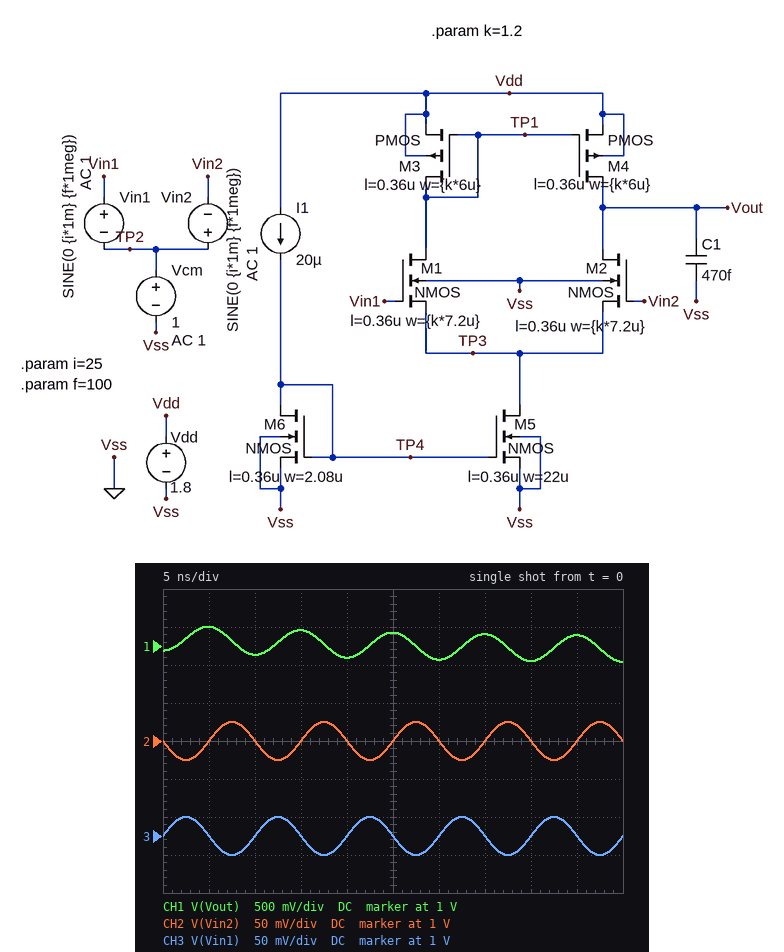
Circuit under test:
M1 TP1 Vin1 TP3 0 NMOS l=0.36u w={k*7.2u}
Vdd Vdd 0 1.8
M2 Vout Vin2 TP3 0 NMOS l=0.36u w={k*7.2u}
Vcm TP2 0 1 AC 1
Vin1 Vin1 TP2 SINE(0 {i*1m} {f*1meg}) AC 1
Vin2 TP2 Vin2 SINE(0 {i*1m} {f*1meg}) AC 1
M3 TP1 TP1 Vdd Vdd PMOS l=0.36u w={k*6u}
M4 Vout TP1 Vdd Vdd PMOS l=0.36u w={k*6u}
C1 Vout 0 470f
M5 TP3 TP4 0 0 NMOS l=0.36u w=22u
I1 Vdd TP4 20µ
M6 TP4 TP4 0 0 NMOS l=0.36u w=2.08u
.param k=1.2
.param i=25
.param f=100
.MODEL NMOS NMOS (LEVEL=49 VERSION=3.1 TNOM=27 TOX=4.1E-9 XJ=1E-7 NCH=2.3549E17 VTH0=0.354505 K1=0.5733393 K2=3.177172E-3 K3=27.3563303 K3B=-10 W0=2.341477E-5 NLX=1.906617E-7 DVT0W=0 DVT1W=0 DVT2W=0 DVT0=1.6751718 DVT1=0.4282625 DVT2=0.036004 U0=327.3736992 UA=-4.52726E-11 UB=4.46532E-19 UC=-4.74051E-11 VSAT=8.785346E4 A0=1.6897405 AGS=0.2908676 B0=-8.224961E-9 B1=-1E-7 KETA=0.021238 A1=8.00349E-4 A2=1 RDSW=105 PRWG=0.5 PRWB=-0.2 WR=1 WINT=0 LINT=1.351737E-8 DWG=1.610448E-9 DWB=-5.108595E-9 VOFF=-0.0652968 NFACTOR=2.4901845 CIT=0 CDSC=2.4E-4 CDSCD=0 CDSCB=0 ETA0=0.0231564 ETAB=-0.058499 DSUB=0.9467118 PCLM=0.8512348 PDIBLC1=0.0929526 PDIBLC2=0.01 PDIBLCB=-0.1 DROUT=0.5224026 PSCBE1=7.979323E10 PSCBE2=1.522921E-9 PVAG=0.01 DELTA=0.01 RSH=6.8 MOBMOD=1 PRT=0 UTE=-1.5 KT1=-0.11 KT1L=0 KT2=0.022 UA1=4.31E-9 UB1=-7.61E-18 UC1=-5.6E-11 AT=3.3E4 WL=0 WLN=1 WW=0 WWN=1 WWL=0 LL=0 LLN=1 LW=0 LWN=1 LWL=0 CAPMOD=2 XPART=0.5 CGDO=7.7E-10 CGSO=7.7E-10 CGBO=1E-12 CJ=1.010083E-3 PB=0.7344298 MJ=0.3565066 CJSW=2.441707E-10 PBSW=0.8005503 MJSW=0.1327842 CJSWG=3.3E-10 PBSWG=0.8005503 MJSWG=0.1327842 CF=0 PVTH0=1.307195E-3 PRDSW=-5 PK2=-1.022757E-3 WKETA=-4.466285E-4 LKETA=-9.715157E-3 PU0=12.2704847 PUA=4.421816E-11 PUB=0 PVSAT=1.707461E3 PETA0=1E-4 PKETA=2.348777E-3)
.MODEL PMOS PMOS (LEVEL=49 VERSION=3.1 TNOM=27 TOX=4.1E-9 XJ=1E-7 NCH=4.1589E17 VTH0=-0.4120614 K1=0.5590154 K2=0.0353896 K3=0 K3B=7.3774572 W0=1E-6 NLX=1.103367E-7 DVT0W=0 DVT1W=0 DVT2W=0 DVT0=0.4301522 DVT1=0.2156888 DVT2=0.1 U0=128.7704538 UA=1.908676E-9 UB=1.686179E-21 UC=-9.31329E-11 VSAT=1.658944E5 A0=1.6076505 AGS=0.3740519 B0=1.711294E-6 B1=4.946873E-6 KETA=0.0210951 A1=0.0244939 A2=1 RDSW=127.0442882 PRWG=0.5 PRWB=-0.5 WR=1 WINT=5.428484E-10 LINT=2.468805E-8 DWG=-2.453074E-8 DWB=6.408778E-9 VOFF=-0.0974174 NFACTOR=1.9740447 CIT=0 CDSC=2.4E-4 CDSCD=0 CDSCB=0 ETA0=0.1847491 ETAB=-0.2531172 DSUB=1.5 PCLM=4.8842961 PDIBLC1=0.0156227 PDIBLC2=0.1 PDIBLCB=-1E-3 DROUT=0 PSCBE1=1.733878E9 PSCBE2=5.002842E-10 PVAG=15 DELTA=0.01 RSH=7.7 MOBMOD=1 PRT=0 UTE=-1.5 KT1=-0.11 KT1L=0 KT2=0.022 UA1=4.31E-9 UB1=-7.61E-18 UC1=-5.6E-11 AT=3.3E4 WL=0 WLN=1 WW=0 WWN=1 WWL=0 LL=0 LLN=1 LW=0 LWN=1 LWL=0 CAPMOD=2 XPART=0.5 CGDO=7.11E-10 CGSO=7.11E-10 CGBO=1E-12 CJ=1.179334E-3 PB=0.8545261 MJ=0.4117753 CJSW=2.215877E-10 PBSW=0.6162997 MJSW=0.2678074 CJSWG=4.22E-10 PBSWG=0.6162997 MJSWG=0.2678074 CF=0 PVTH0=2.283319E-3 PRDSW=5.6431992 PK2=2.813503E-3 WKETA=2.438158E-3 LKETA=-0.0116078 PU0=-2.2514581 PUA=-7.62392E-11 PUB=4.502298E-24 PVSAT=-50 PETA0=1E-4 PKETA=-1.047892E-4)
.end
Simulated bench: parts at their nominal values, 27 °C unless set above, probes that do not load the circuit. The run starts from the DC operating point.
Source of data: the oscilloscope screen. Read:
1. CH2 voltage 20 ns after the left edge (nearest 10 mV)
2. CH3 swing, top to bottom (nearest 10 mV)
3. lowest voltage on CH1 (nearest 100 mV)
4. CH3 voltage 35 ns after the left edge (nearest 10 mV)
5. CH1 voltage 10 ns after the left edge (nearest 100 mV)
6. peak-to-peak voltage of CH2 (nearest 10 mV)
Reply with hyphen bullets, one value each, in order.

- 1.00 V
- 50 mV
- 800 mV
- 1.00 V
- 900 mV
- 50 mV
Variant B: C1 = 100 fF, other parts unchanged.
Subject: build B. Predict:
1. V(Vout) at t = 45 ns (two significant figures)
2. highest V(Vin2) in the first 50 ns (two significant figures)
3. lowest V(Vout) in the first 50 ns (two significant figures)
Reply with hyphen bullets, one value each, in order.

- 1.5 V
- 1.0 V
- 370 mV
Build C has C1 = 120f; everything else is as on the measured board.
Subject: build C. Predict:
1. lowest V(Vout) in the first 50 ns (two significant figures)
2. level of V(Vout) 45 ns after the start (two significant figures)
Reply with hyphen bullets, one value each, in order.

- 410 mV
- 1.5 V
